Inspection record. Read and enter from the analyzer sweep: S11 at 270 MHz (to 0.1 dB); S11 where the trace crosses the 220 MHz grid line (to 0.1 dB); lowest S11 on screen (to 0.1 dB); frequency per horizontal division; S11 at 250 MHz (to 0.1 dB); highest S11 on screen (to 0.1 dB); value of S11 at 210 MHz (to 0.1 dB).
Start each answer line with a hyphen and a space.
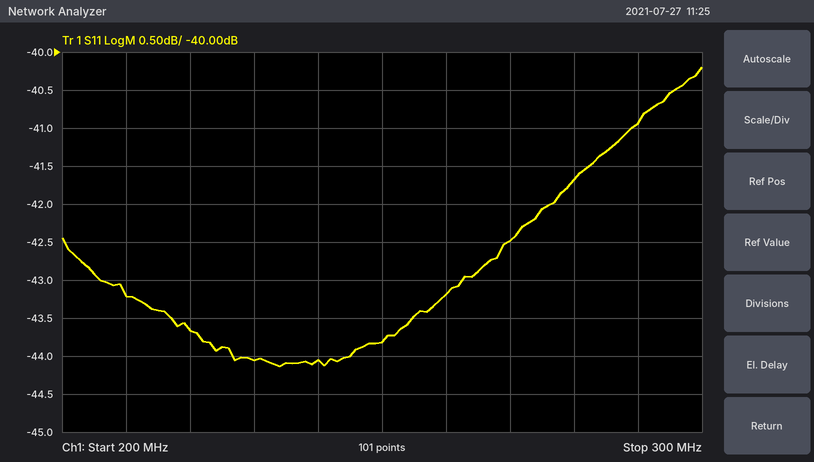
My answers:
- -42.5 dB
- -43.7 dB
- -44.1 dB
- 10 MHz
- -43.8 dB
- -40.2 dB
- -43.2 dB
